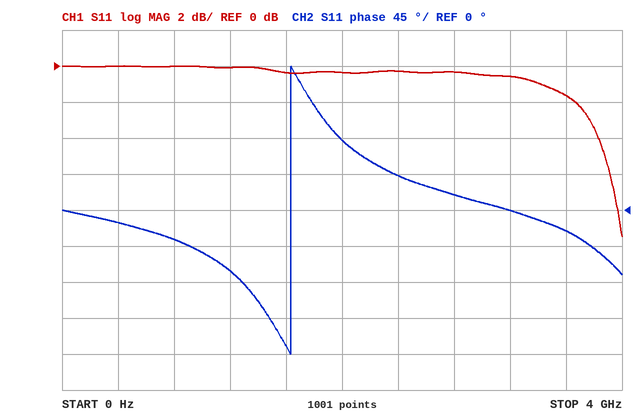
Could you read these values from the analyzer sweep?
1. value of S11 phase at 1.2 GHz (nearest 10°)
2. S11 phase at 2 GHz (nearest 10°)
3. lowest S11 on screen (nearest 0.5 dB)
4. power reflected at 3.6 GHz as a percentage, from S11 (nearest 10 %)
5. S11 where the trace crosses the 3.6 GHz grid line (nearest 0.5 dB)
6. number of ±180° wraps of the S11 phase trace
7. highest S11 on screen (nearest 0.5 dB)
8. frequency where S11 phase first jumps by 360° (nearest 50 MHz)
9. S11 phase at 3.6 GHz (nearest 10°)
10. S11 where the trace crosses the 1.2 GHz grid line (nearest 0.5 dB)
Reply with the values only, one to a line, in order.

-80°
90°
-9.5 dB
70 %
-1.5 dB
1
0.0 dB
1.65 GHz
-30°
0.0 dB
